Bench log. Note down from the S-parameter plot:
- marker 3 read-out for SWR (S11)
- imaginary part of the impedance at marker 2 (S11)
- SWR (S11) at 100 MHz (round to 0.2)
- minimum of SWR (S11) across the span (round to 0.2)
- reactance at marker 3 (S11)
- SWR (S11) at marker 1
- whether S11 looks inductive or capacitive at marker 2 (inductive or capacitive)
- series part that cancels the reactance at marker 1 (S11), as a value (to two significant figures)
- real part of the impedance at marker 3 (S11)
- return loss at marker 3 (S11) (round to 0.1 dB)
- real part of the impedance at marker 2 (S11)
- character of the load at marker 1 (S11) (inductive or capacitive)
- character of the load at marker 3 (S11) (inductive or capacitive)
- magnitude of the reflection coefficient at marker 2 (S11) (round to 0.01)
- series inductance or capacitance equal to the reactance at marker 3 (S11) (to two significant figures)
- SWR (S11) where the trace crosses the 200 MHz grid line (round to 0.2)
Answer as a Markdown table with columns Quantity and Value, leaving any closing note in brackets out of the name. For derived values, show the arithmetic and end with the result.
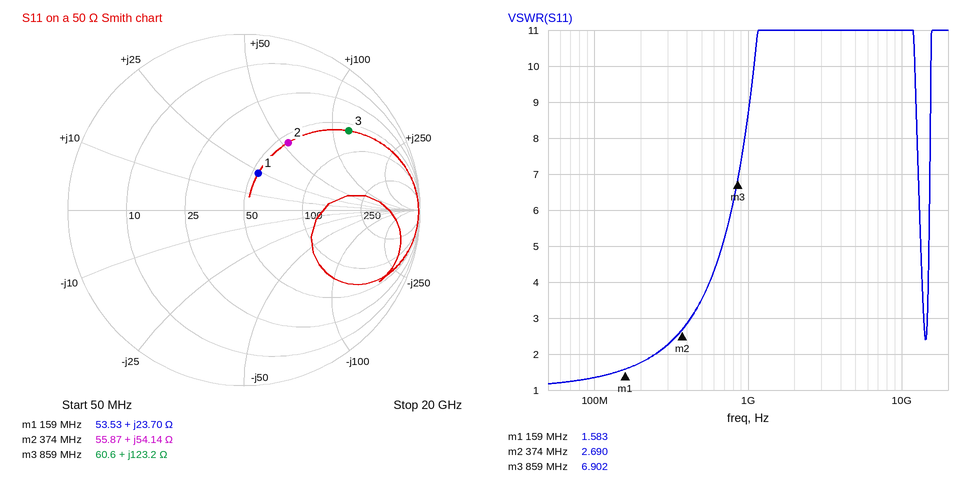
| Quantity | Value |
|---|---|
| marker 3 read-out for SWR | 6.902 |
| imaginary part of the impedance at marker 2 | +54.14 Ω |
| SWR (S11) at 100 MHz | 1.4 |
| minimum of SWR (S11) across the span | 1.2 |
| reactance at marker 3 | +123.2 Ω |
| SWR (S11) at marker 1 | 1.583 |
| whether S11 looks inductive or capacitive at marker 2 | inductive |
| series part that cancels the reactance at marker 1 (S11), as a value | C = 1/(2π × 159 MHz × 23.7 Ω) ≈ 42 pF |
| real part of the impedance at marker 3 | 60.6 Ω |
| return loss at marker 3 (S11) | 2.5 dB |
| real part of the impedance at marker 2 | 55.87 Ω |
| character of the load at marker 1 (S11) | inductive |
| character of the load at marker 3 (S11) | inductive |
| magnitude of the reflection coefficient at marker 2 (S11) | 0.46 |
| series inductance or capacitance equal to the reactance at marker 3 (S11) | L = 123.2 Ω/(2π × 859 MHz) ≈ 23 nH |
| SWR (S11) where the trace crosses the 200 MHz grid line | 1.8 |
